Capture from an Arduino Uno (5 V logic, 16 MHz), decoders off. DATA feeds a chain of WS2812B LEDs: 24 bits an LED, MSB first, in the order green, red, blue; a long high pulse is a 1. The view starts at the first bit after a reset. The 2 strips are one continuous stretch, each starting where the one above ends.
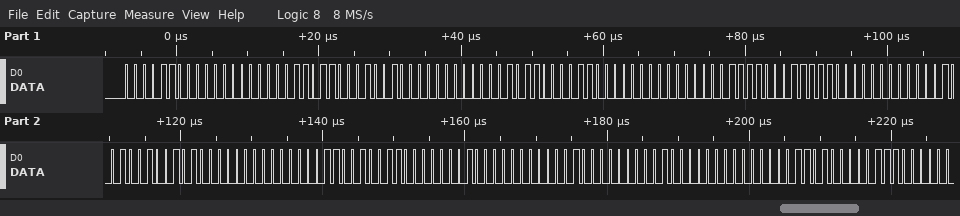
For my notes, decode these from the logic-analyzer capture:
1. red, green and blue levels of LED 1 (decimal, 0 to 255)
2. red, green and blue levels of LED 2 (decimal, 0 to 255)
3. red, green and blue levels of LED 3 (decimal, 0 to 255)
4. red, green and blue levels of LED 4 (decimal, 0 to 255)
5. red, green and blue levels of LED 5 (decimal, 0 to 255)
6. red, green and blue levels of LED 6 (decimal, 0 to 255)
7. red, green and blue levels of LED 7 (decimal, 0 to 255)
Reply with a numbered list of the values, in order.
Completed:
1. 0, 12, 27
2. 0, 18, 22
3. 0, 24, 15
4. 0, 31, 9
5. 0, 37, 3
6. 2, 38, 0
7. 8, 32, 0
